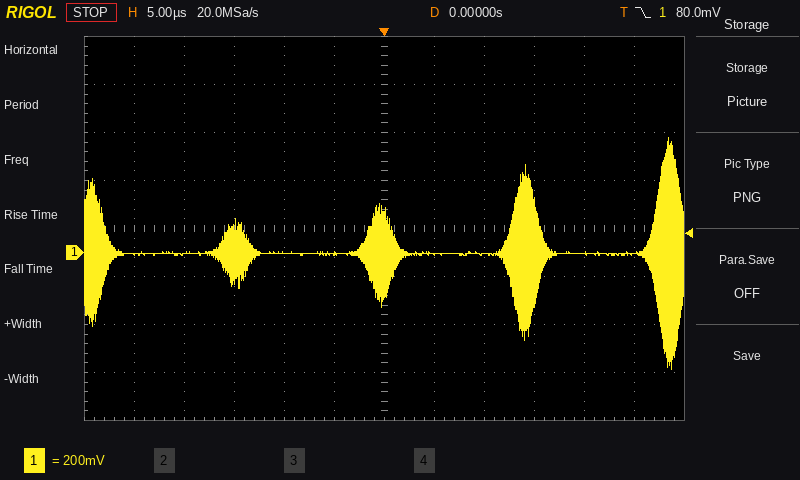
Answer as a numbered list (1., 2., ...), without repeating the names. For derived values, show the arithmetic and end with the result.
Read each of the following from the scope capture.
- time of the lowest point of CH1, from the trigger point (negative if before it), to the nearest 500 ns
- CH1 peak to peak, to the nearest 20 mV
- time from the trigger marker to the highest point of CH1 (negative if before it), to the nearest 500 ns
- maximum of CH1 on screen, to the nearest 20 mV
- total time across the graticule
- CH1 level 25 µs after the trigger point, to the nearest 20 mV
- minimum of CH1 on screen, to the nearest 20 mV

1. +28.5 µs
2. 480 mV − (-480 mV) = 960 mV
3. +28.5 µs
4. 480 mV
5. 60 µs
6. 0 mV
7. -480 mV
